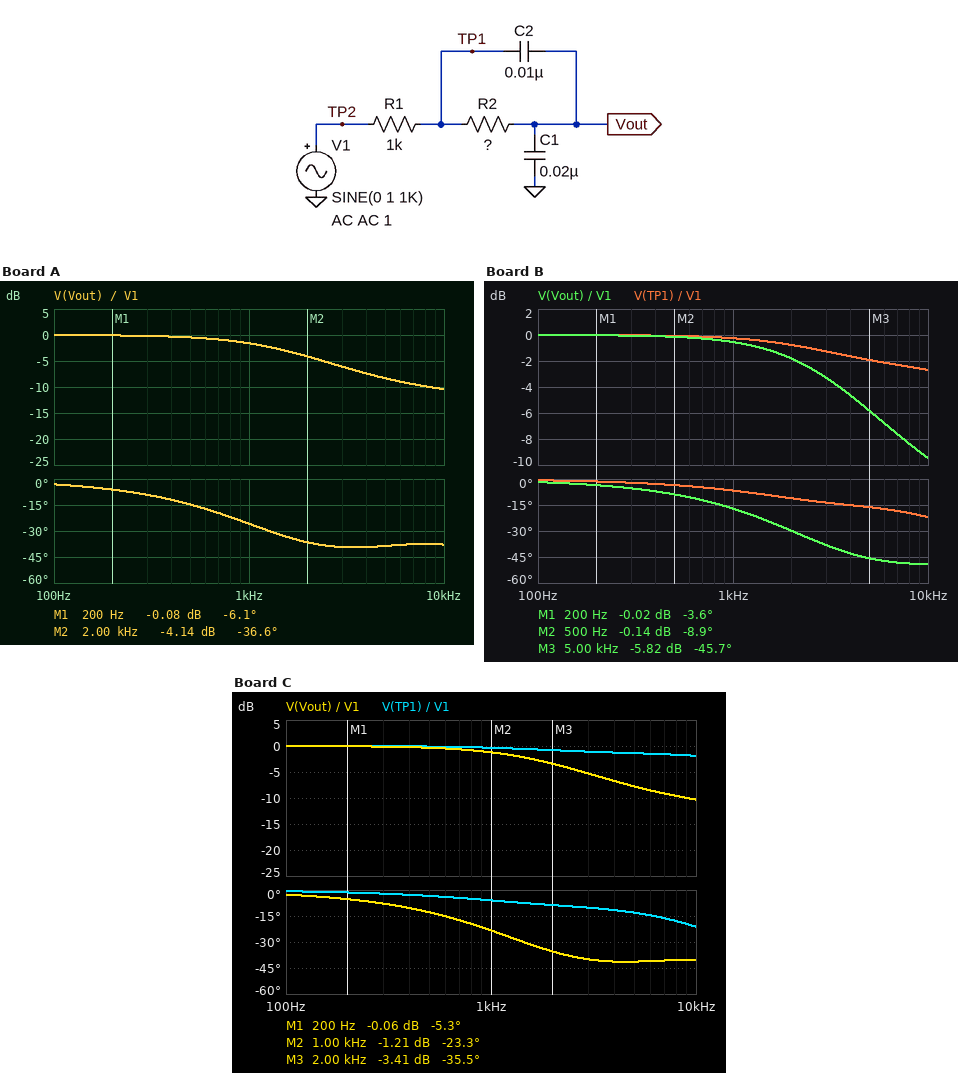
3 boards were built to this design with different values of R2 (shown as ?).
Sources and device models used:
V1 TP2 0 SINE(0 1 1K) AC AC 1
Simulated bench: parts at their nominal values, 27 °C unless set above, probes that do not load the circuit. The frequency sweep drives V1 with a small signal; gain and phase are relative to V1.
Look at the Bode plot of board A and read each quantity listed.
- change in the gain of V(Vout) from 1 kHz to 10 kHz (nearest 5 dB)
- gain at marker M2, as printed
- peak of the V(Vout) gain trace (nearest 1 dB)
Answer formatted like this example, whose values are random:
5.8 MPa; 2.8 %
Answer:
-10 dB; -4.14 dB; 0 dB
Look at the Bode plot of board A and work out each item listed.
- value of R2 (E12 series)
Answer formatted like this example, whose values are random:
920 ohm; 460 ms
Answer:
3.3 kΩ
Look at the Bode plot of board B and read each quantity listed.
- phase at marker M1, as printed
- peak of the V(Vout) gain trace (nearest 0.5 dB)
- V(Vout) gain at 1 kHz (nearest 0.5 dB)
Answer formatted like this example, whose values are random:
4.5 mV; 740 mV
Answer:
-3.6 deg; 0 dB; -0.5 dB
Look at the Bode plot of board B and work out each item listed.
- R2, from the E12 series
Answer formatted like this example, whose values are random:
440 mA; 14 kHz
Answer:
1.5 kΩ
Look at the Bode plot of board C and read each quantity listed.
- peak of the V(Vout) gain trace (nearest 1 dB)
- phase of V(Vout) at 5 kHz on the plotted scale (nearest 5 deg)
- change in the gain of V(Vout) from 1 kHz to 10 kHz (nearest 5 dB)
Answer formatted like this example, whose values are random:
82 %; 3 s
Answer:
0 dB; -40 deg; -10 dB
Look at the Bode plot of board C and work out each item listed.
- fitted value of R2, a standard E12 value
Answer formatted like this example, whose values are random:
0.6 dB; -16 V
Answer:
2.7 kΩ
